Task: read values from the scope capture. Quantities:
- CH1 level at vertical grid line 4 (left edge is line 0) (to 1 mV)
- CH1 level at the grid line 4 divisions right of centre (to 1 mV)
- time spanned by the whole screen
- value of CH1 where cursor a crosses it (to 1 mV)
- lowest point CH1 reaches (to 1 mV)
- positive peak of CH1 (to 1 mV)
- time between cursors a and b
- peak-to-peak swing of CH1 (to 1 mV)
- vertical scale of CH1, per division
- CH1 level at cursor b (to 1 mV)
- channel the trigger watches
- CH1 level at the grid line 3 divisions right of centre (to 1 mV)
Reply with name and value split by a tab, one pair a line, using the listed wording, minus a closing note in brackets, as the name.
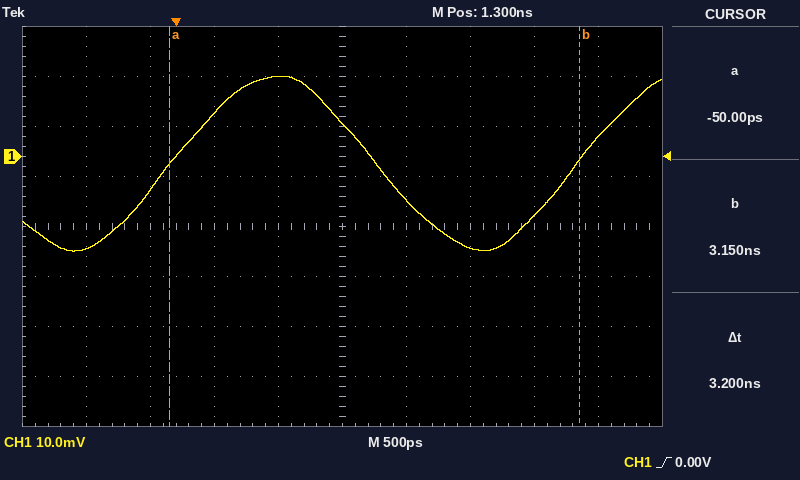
CH1 level at vertical grid line 4 (left edge is line 0)	16 mV
CH1 level at the grid line 4 divisions right of centre	4 mV
time spanned by the whole screen	5 ns
value of CH1 where cursor a crosses it	-1 mV
lowest point CH1 reaches	-19 mV
positive peak of CH1	16 mV
time between cursors a and b	3.2 ns
peak-to-peak swing of CH1	35 mV
vertical scale of CH1, per division	10 mV
CH1 level at cursor b	-1 mV
channel the trigger watches	CH1
CH1 level at the grid line 3 divisions right of centre	-12 mV
